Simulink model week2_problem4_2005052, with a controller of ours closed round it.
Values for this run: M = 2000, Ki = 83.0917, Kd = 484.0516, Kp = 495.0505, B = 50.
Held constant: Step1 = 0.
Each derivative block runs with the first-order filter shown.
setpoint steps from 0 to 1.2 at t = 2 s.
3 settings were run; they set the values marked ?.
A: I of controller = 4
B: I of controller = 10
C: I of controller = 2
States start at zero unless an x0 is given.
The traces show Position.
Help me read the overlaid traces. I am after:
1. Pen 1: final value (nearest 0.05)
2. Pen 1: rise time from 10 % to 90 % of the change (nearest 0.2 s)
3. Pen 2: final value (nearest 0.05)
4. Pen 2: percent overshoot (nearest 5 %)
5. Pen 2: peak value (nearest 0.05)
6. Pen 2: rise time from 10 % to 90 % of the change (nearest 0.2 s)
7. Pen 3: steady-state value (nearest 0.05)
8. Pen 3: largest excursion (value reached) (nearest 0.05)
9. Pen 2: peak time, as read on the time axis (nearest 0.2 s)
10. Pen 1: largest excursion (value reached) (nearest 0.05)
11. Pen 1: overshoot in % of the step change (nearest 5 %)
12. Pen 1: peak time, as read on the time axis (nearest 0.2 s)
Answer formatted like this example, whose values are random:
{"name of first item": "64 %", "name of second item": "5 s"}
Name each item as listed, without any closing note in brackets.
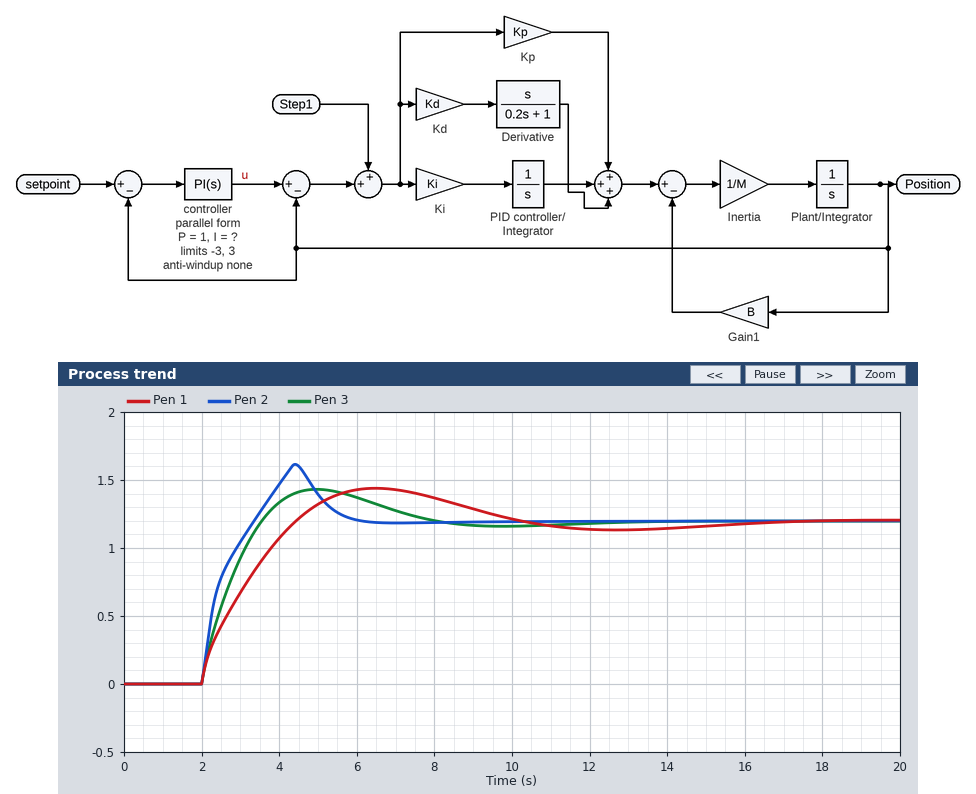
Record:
{"Pen 1: final value": "1.20", "Pen 1: rise time from 10 % to 90 % of the change": "2.0 s", "Pen 2: final value": "1.20", "Pen 2: percent overshoot": "35 %", "Pen 2: peak value": "1.60", "Pen 2: rise time from 10 % to 90 % of the change": "1.0 s", "Pen 3: steady-state value": "1.20", "Pen 3: largest excursion (value reached)": "1.45", "Pen 2: peak time, as read on the time axis": "4.4 s", "Pen 1: largest excursion (value reached)": "1.45", "Pen 1: overshoot in % of the step change": "20 %", "Pen 1: peak time, as read on the time axis": "6.4 s"}
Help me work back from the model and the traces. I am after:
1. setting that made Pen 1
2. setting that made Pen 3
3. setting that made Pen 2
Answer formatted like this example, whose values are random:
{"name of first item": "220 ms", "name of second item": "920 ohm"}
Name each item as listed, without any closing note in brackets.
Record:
{"setting that made Pen 1": "C", "setting that made Pen 3": "A", "setting that made Pen 2": "B"}
